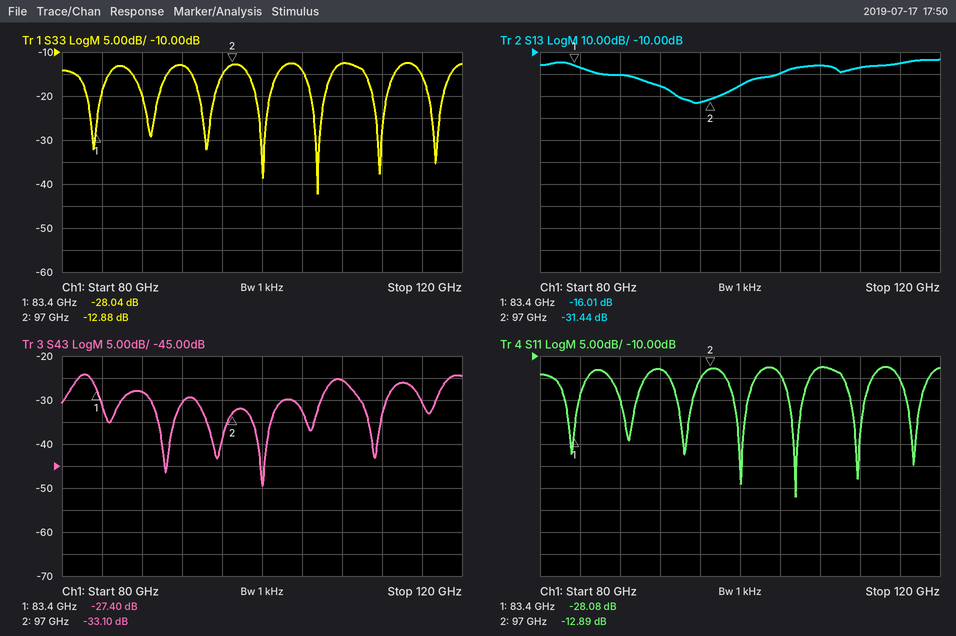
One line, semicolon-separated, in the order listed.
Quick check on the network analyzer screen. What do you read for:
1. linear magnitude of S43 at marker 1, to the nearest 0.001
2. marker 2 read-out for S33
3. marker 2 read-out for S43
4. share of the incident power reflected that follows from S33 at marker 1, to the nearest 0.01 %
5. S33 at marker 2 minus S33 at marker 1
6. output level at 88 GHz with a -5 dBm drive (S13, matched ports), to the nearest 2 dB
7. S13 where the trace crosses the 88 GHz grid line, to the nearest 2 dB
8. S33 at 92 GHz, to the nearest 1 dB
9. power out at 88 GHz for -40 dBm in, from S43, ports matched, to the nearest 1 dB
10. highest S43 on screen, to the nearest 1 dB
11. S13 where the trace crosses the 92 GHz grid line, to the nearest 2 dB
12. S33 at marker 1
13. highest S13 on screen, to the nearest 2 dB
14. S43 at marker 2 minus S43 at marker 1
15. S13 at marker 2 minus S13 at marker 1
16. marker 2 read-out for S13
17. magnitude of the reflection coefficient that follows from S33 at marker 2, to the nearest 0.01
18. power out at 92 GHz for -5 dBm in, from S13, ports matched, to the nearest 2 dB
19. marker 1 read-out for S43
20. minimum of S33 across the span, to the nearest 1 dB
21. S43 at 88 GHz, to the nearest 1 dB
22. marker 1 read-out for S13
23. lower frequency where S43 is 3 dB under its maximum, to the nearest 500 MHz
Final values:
0.043; -12.88 dB; -33.10 dB; 0.16 %; 15.16 dB; -26 dBm; -20 dB; -13 dB; -68 dBm; -24 dB; -26 dB; -28.04 dB; -14 dB; -5.70 dB; -15.43 dB; -31.44 dB; 0.23; -30 dBm; -27.40 dB; -42 dB; -28 dB; -16.01 dB; 81.0 GHz
